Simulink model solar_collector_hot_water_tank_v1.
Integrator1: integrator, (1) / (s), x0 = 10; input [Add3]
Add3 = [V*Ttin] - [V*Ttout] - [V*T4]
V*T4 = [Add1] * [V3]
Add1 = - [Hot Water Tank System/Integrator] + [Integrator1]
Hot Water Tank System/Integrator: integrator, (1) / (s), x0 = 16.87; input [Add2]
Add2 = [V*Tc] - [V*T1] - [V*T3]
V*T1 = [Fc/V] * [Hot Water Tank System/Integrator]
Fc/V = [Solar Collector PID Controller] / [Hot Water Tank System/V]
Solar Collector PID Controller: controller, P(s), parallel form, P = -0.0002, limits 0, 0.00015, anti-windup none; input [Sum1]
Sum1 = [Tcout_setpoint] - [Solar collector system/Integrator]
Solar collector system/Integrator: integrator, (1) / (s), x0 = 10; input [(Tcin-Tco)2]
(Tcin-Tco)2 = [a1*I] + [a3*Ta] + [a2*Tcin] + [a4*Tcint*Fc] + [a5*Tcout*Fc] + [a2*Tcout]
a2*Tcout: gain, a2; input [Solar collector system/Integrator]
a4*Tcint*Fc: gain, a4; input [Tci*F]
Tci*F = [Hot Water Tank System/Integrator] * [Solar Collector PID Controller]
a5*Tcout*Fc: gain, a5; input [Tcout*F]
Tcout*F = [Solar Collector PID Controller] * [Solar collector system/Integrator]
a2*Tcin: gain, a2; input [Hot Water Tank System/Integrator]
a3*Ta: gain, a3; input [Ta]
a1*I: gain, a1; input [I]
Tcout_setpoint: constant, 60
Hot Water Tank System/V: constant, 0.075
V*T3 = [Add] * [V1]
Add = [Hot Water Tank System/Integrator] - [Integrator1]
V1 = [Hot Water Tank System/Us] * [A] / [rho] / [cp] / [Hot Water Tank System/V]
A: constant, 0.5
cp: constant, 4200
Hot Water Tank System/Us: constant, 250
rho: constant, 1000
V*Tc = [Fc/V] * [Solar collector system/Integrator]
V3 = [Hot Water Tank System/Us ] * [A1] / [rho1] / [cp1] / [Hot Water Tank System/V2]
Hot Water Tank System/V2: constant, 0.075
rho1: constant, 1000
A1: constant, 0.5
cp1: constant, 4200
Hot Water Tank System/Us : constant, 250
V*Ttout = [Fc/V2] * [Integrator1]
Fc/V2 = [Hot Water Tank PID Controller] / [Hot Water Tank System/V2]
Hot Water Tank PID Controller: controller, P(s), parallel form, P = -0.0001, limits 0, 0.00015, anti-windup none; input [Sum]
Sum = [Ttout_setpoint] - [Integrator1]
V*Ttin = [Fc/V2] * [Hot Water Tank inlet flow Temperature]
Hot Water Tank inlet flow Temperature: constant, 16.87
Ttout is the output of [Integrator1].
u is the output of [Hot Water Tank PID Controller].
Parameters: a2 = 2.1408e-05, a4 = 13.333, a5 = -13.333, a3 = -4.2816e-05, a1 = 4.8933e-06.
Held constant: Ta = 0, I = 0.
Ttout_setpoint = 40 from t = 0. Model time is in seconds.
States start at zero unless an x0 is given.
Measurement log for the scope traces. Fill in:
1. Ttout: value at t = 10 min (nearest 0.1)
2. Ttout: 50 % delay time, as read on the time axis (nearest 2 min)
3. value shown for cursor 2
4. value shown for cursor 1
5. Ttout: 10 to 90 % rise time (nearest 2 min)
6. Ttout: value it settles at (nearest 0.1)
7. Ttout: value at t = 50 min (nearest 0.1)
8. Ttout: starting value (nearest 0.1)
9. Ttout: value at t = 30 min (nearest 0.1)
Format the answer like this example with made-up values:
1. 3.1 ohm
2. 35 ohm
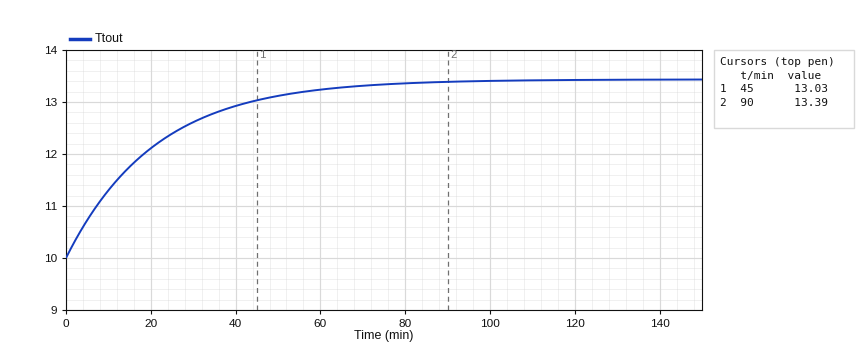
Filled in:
1. 11.3
2. 14 min
3. 13.39
4. 13.03
5. 46 min
6. 13.4
7. 13.1
8. 10.0
9. 12.6
